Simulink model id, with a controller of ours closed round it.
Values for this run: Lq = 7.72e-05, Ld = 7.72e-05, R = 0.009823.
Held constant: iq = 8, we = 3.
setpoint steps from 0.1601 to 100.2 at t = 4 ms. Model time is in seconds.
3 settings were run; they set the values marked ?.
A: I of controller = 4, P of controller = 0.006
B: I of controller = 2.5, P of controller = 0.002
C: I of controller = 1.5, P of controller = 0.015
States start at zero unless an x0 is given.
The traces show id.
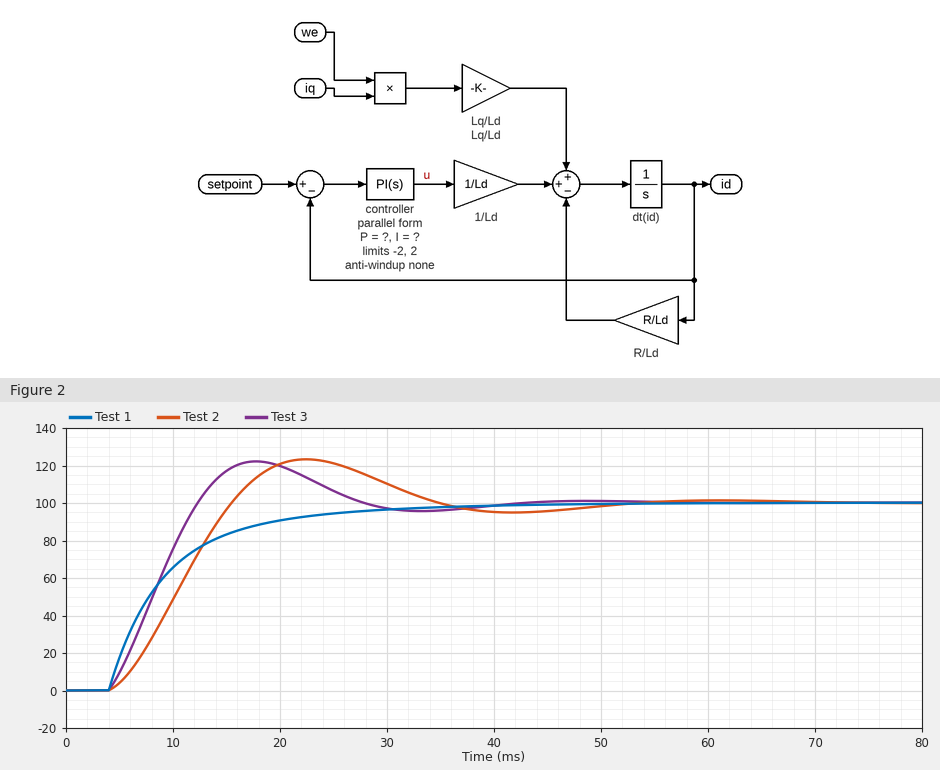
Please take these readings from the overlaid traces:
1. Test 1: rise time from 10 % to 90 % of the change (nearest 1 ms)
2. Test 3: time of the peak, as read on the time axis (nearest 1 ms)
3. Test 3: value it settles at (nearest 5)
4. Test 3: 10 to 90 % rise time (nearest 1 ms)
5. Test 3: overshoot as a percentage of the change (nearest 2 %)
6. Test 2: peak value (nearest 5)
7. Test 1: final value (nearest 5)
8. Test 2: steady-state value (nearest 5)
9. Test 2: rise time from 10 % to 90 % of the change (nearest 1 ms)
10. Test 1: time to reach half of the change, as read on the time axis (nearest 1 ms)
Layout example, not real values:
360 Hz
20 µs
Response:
15 ms
18 ms
100
6 ms
22 %
125
100
100
8 ms
8 ms
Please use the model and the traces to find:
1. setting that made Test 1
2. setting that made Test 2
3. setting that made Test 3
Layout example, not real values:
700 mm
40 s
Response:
C
B
A
